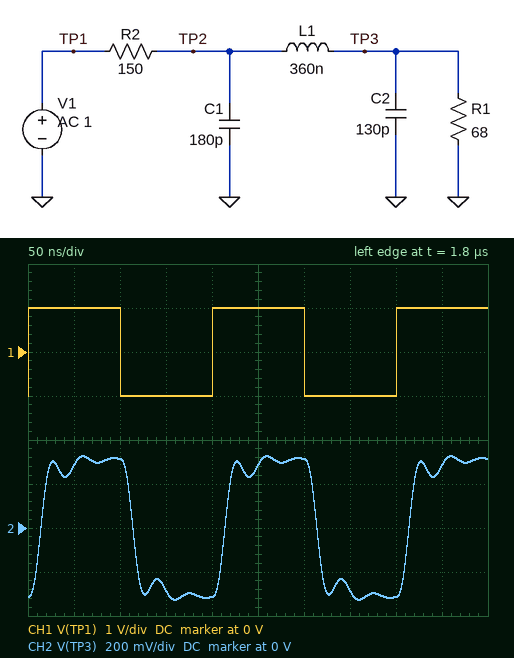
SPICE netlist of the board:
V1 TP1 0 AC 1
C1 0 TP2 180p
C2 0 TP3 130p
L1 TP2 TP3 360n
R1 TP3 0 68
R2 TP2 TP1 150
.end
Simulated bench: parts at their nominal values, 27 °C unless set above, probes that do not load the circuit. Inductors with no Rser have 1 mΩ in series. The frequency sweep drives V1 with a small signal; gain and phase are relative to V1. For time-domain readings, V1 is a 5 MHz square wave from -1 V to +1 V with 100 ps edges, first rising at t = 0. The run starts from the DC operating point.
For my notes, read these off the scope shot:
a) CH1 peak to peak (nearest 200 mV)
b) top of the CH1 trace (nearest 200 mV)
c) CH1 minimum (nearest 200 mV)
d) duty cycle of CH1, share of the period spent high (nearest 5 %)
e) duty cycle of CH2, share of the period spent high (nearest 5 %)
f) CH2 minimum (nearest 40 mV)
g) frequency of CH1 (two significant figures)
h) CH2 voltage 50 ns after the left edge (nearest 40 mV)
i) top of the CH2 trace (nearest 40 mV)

2.0 V
1.0 V
-1.0 V
50 %
50 %
-320 mV
5.0 MHz
280 mV
320 mV
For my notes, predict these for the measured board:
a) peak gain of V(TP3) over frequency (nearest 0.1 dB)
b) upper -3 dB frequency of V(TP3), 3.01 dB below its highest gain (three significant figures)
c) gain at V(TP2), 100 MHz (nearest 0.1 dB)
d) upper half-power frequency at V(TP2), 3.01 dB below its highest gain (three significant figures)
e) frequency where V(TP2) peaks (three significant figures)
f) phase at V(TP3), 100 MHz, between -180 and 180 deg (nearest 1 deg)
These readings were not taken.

-10.1 dB
32.1 MHz
-24.2 dB
38.6 MHz
30.4 MHz
104 deg
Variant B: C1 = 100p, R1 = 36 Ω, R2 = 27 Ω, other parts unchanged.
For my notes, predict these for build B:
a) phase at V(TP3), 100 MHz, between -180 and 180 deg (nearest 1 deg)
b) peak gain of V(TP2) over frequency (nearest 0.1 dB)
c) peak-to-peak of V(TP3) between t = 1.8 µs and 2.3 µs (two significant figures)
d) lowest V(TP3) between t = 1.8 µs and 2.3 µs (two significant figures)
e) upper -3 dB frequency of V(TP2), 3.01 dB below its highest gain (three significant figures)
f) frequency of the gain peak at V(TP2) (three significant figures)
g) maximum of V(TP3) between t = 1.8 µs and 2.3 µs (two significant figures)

142 deg
-1.0 dB
1.3 V
-630 mV
81.5 MHz
38.9 MHz
630 mV
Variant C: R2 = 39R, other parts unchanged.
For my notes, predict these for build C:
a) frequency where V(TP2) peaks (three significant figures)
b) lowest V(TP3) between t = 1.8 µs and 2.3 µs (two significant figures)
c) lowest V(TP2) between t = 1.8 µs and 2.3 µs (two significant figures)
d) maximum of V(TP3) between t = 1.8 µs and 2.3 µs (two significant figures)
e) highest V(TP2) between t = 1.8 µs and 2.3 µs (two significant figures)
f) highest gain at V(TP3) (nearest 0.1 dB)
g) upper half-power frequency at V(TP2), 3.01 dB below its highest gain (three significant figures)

32.7 MHz
-780 mV
-680 mV
780 mV
680 mV
-3.7 dB
49.4 MHz
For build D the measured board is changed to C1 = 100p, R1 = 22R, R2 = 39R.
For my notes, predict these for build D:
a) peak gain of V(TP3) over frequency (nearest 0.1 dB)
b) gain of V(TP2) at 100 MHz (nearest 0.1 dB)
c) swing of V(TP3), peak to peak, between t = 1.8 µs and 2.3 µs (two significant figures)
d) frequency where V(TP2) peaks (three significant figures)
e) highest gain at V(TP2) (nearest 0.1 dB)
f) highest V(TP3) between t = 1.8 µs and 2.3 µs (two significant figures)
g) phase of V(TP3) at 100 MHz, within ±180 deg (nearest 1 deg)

-8.9 dB
-7.9 dB
790 mV
34.0 MHz
-1.3 dB
390 mV
144 deg
